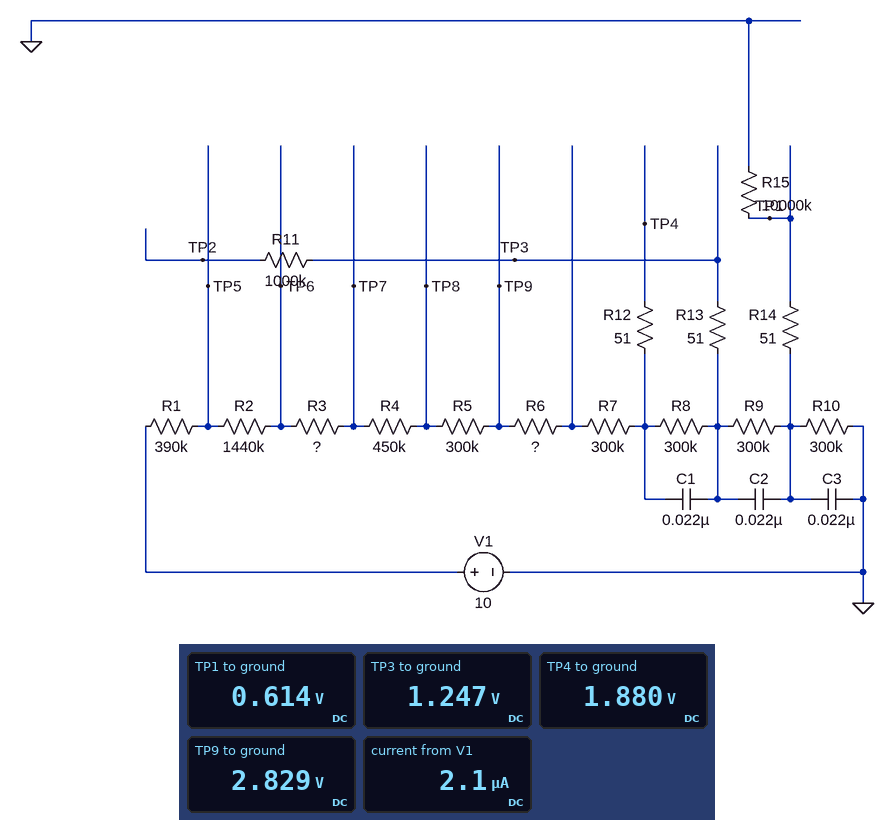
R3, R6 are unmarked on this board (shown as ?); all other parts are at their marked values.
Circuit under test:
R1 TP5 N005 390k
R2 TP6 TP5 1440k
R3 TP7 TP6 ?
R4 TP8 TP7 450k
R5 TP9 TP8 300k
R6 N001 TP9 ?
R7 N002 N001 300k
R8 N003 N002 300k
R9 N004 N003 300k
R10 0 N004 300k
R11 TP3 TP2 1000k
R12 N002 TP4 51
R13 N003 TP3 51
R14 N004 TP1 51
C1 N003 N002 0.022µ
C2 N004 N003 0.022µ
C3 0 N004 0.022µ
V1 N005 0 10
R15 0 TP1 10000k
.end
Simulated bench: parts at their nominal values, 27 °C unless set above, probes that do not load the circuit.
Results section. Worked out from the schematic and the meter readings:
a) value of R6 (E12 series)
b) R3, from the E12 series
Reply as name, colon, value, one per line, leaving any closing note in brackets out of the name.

value of R6: 150 kΩ
R3, from the E12 series: 820 kΩ
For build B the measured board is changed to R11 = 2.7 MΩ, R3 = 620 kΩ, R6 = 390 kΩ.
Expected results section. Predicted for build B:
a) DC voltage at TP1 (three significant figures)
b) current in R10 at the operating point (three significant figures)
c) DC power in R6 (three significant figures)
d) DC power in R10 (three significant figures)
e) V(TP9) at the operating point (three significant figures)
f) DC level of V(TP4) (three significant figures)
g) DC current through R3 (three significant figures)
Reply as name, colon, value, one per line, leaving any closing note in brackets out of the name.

DC voltage at TP1: 609 mV
current in R10 at the operating point: 2.03 µA
DC power in R6: 1.71 µW
DC power in R10: 1.24 µW
V(TP9) at the operating point: 3.31 V
DC level of V(TP4): 1.86 V
DC current through R3: 2.09 µA
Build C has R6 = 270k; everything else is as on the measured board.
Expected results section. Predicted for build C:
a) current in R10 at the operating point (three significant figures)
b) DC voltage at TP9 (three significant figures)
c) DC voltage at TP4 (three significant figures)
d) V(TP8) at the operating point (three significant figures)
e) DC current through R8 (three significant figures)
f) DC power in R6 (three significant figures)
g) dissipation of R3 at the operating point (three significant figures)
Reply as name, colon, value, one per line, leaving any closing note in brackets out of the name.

current in R10 at the operating point: 2.00 µA
DC voltage at TP9: 3.01 V
DC voltage at TP4: 1.83 V
V(TP8) at the operating point: 3.62 V
DC current through R8: 2.06 µA
DC power in R6: 1.14 µW
dissipation of R3 at the operating point: 3.47 µW
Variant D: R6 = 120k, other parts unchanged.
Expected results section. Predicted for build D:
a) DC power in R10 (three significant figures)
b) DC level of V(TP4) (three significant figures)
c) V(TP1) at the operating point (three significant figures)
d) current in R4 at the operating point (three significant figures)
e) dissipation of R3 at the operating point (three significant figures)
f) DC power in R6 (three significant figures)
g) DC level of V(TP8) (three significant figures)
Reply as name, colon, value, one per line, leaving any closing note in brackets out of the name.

DC power in R10: 1.27 µW
DC level of V(TP4): 1.89 V
V(TP1) at the operating point: 618 mV
current in R4 at the operating point: 2.12 µA
dissipation of R3 at the operating point: 3.69 µW
DC power in R6: 541 nW
DC level of V(TP8): 3.42 V
